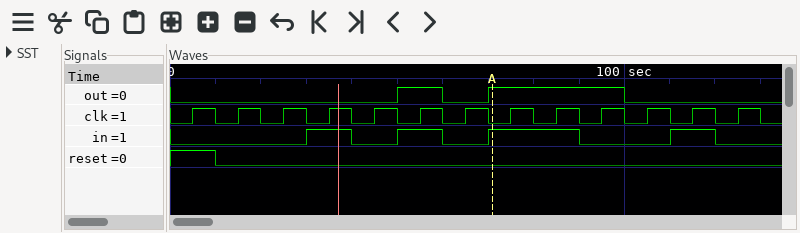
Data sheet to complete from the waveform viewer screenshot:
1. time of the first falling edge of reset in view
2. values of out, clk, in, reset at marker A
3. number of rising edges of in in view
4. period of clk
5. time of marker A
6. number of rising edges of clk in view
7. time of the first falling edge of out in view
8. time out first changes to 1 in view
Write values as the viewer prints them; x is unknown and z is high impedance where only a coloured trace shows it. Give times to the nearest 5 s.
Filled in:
10 s
out=1, clk=0, in=1, reset=0
4
10 s
70 s
13
60 s
50 s
